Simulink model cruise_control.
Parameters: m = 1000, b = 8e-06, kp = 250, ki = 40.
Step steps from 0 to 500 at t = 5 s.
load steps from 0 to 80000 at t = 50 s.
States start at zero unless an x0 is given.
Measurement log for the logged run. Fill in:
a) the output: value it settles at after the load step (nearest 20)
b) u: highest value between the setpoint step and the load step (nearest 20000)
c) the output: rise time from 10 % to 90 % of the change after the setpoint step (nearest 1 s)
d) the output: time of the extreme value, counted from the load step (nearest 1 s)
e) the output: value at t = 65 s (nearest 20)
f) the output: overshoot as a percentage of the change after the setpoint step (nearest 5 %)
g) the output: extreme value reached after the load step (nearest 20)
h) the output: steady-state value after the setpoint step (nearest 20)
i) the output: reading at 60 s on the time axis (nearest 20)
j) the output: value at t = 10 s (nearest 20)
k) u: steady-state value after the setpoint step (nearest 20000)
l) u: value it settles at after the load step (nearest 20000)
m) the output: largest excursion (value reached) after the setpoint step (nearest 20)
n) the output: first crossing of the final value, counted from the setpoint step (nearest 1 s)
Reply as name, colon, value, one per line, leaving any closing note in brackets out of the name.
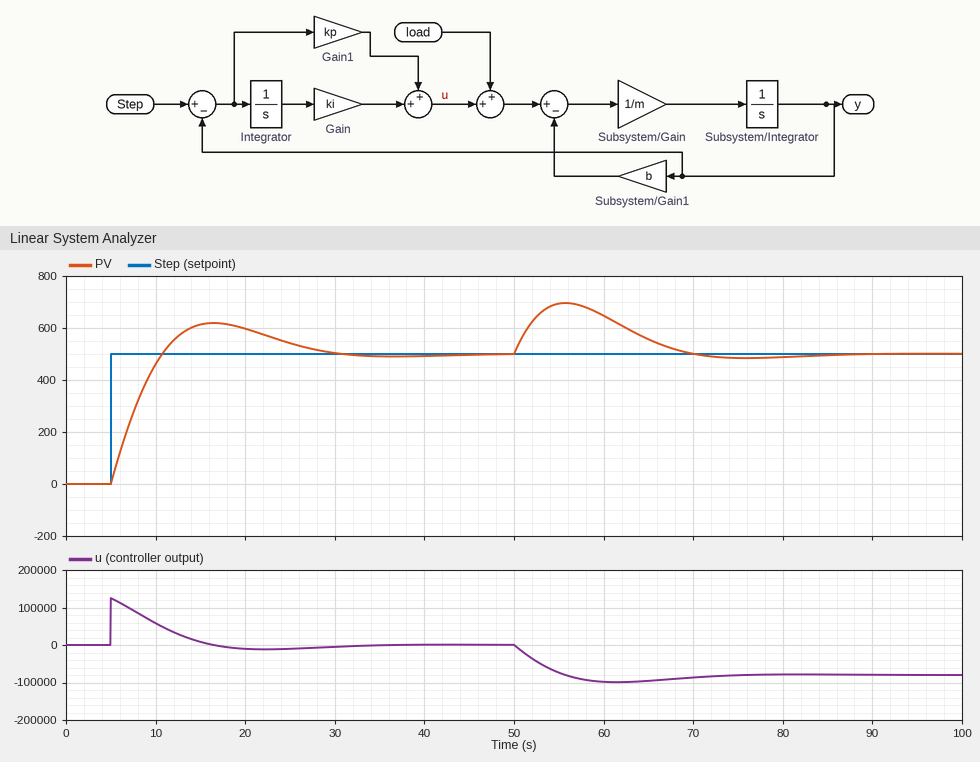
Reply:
the output: value it settles at after the load step: 500
u: highest value between the setpoint step and the load step: 120000
the output: rise time from 10 % to 90 % of the change after the setpoint step: 4 s
the output: time of the extreme value, counted from the load step: 6 s
the output: value at t = 65 s: 560
the output: overshoot as a percentage of the change after the setpoint step: 25 %
the output: extreme value reached after the load step: 700
the output: steady-state value after the setpoint step: 500
the output: reading at 60 s on the time axis: 640
the output: value at t = 10 s: 460
u: steady-state value after the setpoint step: 0
u: value it settles at after the load step: -80000
the output: largest excursion (value reached) after the setpoint step: 620
the output: first crossing of the final value, counted from the setpoint step: 6 s
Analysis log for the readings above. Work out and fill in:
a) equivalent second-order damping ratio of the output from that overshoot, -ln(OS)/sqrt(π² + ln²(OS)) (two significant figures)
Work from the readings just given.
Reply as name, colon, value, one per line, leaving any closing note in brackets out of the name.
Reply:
equivalent second-order damping ratio of the output from that overshoot, -ln(OS)/sqrt(π² + ln²(OS)): 0.40
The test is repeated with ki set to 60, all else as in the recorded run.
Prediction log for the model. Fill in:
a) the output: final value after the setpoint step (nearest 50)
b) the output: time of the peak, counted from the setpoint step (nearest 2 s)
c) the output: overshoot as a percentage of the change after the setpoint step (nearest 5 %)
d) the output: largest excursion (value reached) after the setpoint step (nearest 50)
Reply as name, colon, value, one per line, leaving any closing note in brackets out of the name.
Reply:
the output: final value after the setpoint step: 500
the output: time of the peak, counted from the setpoint step: 10 s
the output: overshoot as a percentage of the change after the setpoint step: 30 %
the output: largest excursion (value reached) after the setpoint step: 650
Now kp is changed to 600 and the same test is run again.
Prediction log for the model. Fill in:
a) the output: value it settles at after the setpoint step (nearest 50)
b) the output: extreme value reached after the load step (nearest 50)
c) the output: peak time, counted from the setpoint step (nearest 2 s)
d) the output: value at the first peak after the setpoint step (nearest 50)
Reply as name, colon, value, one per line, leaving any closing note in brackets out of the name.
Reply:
the output: value it settles at after the setpoint step: 500
the output: extreme value reached after the load step: 600
the output: peak time, counted from the setpoint step: 8 s
the output: value at the first peak after the setpoint step: 550
